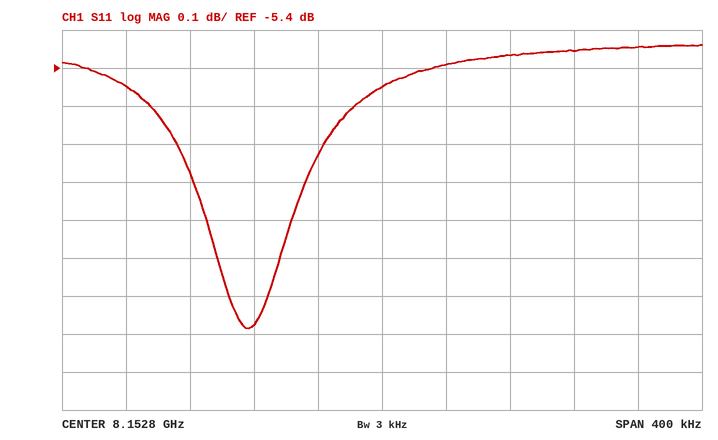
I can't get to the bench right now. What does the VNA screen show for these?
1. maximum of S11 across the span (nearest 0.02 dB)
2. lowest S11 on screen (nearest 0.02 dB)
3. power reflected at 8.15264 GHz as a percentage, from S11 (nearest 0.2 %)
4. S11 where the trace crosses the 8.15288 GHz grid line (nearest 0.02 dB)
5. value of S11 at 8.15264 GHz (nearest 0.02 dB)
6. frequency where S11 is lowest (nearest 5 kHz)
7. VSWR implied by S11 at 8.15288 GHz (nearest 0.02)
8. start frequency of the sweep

-5.34 dB
-6.08 dB
28.6 %
-5.36 dB
-5.44 dB
8.152715 GHz
3.34
8.1526 GHz
